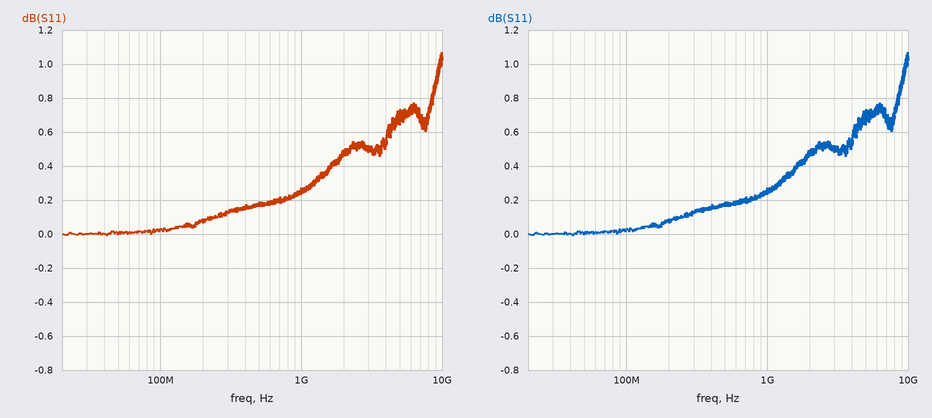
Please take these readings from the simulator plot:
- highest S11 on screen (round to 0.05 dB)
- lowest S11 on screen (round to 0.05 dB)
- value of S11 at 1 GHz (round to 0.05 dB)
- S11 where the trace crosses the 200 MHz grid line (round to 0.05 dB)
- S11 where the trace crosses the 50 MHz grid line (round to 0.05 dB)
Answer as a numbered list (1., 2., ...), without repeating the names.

1. 1.05 dB
2. 0.00 dB
3. 0.25 dB
4. 0.10 dB
5. 0.00 dB
